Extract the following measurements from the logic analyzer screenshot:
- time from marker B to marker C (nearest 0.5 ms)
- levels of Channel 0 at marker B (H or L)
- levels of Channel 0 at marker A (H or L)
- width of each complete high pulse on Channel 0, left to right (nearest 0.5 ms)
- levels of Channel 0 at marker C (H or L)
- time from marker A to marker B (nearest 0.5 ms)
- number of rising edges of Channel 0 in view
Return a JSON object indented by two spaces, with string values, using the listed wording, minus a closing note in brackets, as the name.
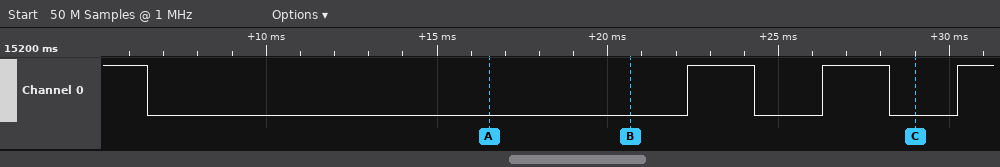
{
  "time from marker B to marker C": "8.5 ms",
  "levels of Channel 0 at marker B": "Channel 0=L",
  "levels of Channel 0 at marker A": "Channel 0=L",
  "width of each complete high pulse on Channel 0, left to right": "2 ms, 2 ms",
  "levels of Channel 0 at marker C": "Channel 0=L",
  "time from marker A to marker B": "4 ms",
  "number of rising edges of Channel 0 in view": "3"
}
